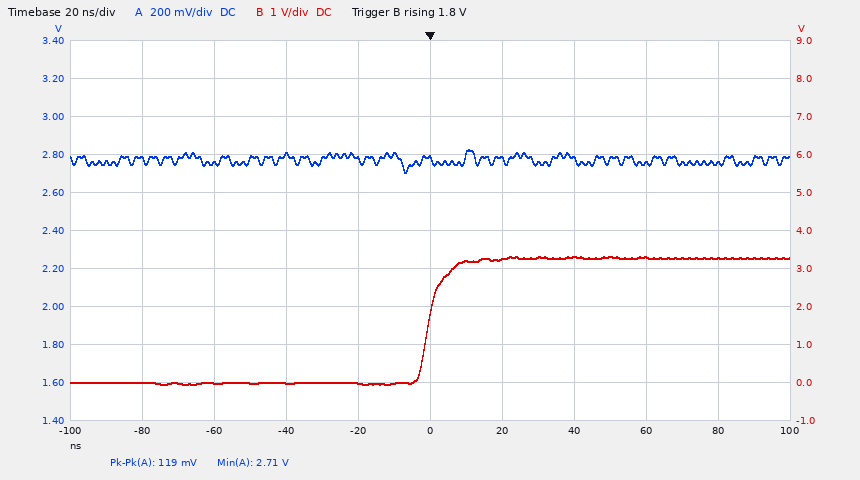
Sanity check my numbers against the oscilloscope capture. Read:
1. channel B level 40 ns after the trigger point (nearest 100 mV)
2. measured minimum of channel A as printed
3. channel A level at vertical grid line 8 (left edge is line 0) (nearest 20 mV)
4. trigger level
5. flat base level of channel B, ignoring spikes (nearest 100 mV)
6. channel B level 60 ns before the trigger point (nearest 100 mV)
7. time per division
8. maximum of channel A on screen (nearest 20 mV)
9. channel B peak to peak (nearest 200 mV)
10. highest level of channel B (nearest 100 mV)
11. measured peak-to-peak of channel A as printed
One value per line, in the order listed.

3.3 V
2.71 V
2.76 V
1.8 V
0.0 V
0.0 V
20 ns
2.82 V
3.4 V
3.3 V
119 mV
